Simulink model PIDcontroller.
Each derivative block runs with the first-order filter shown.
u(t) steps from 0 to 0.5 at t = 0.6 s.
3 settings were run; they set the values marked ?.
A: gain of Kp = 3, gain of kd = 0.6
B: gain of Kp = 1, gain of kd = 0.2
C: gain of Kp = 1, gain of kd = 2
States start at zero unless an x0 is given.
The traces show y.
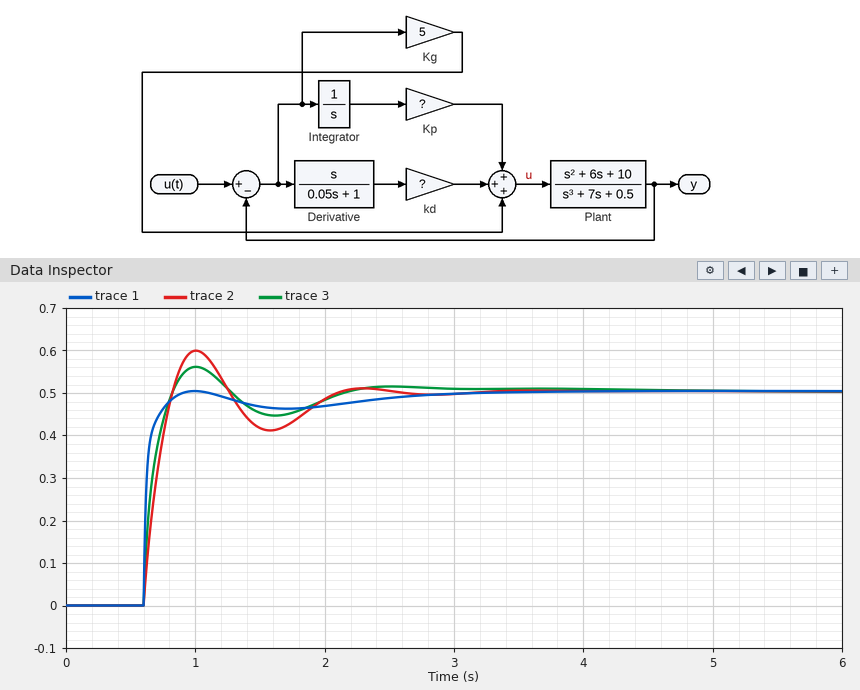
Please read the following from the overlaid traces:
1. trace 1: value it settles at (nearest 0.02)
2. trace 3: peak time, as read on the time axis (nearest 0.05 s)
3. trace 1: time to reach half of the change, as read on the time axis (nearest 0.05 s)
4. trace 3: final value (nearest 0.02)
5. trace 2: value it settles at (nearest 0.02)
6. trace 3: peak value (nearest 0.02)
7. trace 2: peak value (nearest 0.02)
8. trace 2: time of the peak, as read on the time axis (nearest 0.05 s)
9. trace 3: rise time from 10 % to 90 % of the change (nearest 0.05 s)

0.50
1.00 s
0.60 s
0.50
0.50
0.56
0.60
1.00 s
0.15 s
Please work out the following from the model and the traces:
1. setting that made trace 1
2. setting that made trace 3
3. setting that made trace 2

C
A
B
